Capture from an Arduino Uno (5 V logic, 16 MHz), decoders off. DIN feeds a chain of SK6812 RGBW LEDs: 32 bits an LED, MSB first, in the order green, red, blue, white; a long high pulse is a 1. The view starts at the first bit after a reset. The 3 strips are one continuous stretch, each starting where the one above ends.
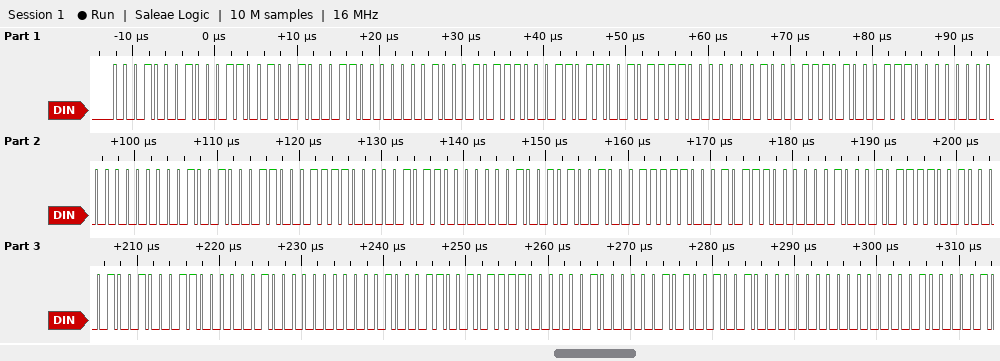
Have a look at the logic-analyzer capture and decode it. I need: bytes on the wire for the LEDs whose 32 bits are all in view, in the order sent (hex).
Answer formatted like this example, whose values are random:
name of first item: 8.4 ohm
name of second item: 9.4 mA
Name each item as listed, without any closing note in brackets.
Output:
bytes on the wire for the LEDs whose 32 bits are all in view, in the order sent: 11 19 23 01 17 1B 2F 01 1D 1C 00 01 23 1E 0B 01 29 1F 17 02 2F 21 23 02 00 23 2F 02 05 24 00 02
